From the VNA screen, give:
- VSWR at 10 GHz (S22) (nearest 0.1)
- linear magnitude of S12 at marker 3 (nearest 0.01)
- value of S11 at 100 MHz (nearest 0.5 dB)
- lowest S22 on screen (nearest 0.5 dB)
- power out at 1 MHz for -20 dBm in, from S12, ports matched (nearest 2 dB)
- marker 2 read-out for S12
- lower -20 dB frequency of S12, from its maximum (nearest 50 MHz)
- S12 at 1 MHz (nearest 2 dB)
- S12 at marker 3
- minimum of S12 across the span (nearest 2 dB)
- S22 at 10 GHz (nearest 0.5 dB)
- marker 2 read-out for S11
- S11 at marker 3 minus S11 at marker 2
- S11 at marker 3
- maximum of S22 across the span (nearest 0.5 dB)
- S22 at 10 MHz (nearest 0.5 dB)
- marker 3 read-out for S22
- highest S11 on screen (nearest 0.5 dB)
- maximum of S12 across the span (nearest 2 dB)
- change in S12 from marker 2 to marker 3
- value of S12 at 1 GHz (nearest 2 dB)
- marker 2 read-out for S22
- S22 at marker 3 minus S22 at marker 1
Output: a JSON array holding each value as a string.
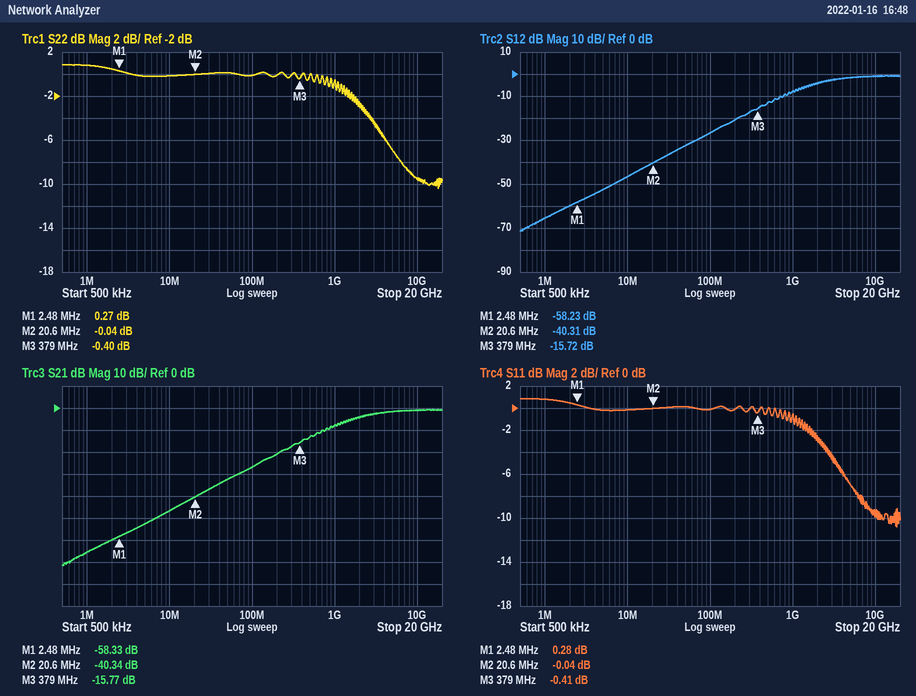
["2.0", "0.16", "0.0 dB", "-10.5 dB", "-86 dBm", "-40.31 dB", "200 MHz", "-66 dB", "-15.72 dB", "-72 dB", "-9.5 dB", "-0.04 dB", "-0.37 dB", "-0.41 dB", "1.0 dB", "0.0 dB", "-0.40 dB", "1.0 dB", "0 dB", "24.59 dB", "-8 dB", "-0.04 dB", "-0.67 dB"]
